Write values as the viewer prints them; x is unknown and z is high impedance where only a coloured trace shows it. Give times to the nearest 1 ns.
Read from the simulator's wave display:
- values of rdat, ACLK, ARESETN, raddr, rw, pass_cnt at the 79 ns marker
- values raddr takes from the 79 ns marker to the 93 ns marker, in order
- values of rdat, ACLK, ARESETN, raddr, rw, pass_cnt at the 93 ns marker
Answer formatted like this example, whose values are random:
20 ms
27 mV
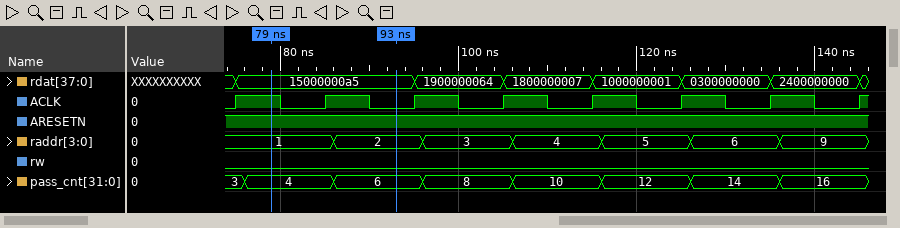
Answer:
rdat=15000000a5, ACLK=1, ARESETN=1, raddr=1, rw=0, pass_cnt=4
1, 2
rdat=15000000a5, ACLK=0, ARESETN=1, raddr=2, rw=0, pass_cnt=6
